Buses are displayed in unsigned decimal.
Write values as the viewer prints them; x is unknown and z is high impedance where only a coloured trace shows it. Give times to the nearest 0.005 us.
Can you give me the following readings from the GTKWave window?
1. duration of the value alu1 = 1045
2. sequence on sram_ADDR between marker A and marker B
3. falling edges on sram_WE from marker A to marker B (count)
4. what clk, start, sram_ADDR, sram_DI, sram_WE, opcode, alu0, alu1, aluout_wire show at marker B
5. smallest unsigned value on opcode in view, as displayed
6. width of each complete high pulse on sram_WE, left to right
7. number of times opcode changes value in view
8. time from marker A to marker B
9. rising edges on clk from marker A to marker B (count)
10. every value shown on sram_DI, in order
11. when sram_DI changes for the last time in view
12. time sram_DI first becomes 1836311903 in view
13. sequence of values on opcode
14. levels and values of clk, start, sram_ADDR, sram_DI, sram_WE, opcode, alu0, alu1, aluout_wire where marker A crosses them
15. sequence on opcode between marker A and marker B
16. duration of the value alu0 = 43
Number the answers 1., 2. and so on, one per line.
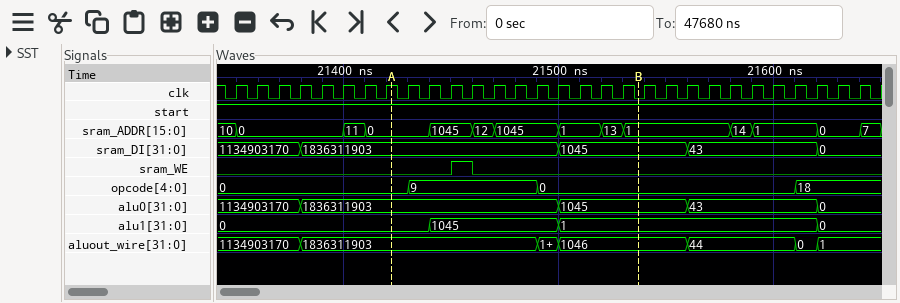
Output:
1. 0.06 us
2. 0, 1045, 12, 1045, 1, 13, 1
3. 1
4. clk=0, start=1, sram_ADDR=1, sram_DI=1045, sram_WE=0, opcode=0, alu0=1045, alu1=1, aluout_wire=1046
5. 0
6. 0.01 us
7. 3
8. 0.115 us
9. 11
10. 1134903170, 1836311903, 1045, 43, 0
11. 21.62 us
12. 21.38 us
13. 0, 9, 0, 18
14. clk=1, start=1, sram_ADDR=0, sram_DI=1836311903, sram_WE=0, opcode=0, alu0=1836311903, alu1=0, aluout_wire=1836311903
15. 0, 9, 0
16. 0.06 us
